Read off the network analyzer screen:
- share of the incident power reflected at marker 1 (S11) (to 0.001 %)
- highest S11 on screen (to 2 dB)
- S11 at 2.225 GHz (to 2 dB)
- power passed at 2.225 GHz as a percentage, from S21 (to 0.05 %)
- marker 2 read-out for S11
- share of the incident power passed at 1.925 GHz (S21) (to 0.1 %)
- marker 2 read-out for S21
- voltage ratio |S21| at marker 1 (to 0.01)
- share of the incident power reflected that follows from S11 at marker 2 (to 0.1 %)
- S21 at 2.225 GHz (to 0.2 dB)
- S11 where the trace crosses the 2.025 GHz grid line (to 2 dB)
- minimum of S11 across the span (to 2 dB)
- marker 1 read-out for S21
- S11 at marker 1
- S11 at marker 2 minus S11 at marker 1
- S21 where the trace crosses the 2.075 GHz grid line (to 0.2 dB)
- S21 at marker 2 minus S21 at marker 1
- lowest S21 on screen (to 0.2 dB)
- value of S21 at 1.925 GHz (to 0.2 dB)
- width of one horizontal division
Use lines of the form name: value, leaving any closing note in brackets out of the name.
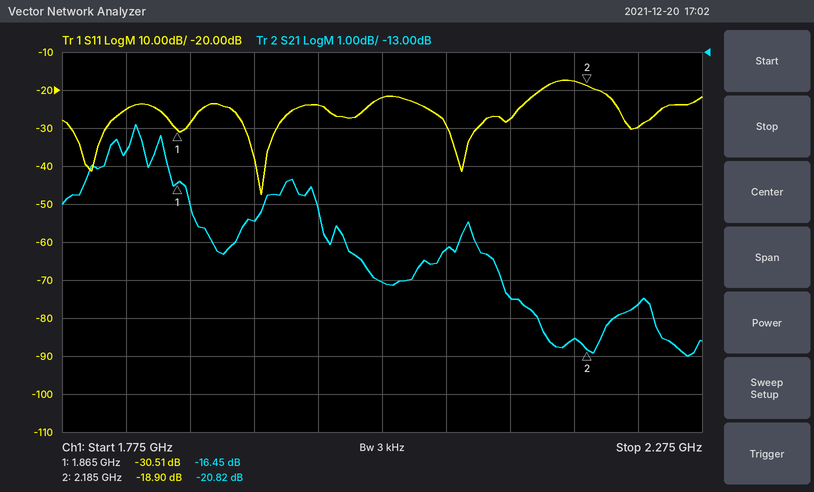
share of the incident power reflected at marker 1 (S11): 0.089 %
highest S11 on screen: -18 dB
S11 at 2.225 GHz: -30 dB
power passed at 2.225 GHz as a percentage, from S21: 1.10 %
marker 2 read-out for S11: -18.90 dB
share of the incident power passed at 1.925 GHz (S21): 1.8 %
marker 2 read-out for S21: -20.82 dB
voltage ratio |S21| at marker 1: 0.15
share of the incident power reflected that follows from S11 at marker 2: 1.3 %
S21 at 2.225 GHz: -19.6 dB
S11 where the trace crosses the 2.025 GHz grid line: -22 dB
minimum of S11 across the span: -48 dB
marker 1 read-out for S21: -16.45 dB
S11 at marker 1: -30.51 dB
S11 at marker 2 minus S11 at marker 1: 11.61 dB
S21 where the trace crosses the 2.075 GHz grid line: -18.2 dB
S21 at marker 2 minus S21 at marker 1: -4.37 dB
lowest S21 on screen: -21.0 dB
value of S21 at 1.925 GHz: -17.4 dB
width of one horizontal division: 50 MHz
